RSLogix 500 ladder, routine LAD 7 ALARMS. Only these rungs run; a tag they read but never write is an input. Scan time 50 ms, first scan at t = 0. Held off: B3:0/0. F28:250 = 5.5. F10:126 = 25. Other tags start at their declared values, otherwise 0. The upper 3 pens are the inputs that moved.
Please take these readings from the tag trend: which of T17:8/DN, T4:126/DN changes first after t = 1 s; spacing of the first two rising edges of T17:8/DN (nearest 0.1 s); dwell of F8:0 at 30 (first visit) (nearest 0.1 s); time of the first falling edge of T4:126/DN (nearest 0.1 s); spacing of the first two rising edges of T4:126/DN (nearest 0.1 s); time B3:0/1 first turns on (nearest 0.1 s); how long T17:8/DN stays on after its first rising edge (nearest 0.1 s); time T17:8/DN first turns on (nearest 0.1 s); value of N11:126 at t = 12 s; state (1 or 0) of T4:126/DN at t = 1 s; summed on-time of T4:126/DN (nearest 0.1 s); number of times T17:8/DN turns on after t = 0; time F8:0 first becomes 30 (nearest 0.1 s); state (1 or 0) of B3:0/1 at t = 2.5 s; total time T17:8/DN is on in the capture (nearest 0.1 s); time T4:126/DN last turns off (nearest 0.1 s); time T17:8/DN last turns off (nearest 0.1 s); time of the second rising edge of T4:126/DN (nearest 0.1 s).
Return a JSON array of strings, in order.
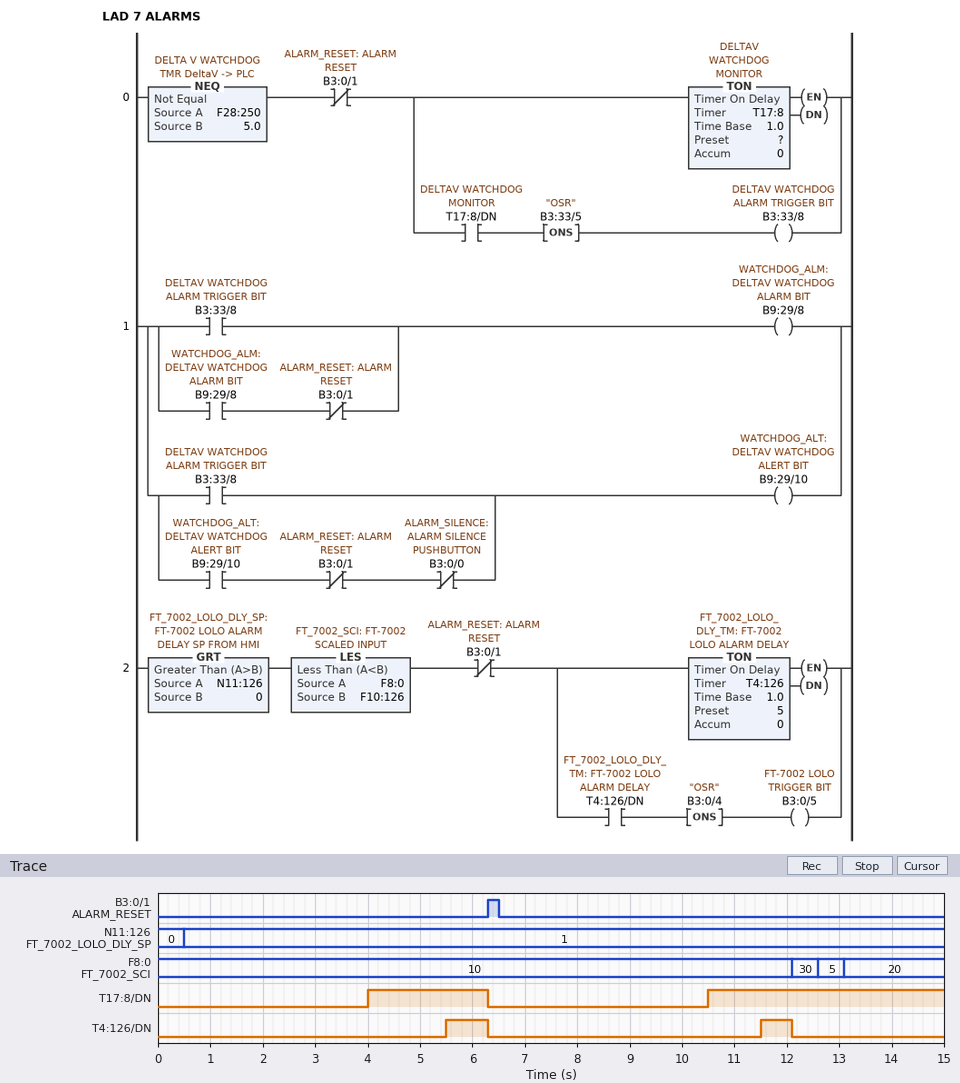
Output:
["T17:8/DN", "6.5 s", "0.5 s", "6.3 s", "6.0 s", "6.3 s", "2.3 s", "4.0 s", "1", "0", "1.4 s", "2", "12.1 s", "0", "6.8 s", "12.1 s", "6.3 s", "11.5 s"]
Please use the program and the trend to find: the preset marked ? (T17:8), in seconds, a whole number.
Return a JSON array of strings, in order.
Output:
["4 s"]
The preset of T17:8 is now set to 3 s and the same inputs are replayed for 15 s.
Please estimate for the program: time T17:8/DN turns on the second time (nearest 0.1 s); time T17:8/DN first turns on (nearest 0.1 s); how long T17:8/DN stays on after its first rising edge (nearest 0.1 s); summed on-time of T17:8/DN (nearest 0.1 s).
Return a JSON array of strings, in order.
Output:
["9.5 s", "3.0 s", "3.3 s", "8.8 s"]
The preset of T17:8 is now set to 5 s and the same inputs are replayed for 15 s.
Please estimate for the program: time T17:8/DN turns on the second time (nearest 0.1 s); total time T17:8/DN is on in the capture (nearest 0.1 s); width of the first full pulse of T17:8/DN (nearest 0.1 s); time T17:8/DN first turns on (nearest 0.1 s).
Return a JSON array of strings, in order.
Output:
["11.5 s", "4.8 s", "1.3 s", "5.0 s"]
